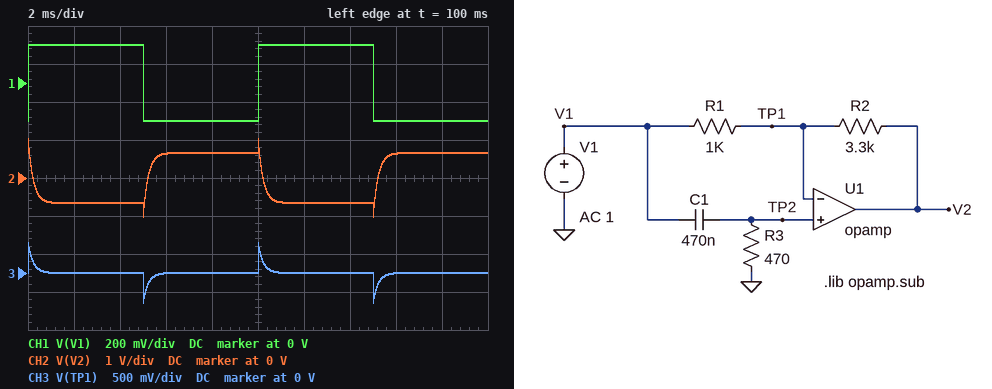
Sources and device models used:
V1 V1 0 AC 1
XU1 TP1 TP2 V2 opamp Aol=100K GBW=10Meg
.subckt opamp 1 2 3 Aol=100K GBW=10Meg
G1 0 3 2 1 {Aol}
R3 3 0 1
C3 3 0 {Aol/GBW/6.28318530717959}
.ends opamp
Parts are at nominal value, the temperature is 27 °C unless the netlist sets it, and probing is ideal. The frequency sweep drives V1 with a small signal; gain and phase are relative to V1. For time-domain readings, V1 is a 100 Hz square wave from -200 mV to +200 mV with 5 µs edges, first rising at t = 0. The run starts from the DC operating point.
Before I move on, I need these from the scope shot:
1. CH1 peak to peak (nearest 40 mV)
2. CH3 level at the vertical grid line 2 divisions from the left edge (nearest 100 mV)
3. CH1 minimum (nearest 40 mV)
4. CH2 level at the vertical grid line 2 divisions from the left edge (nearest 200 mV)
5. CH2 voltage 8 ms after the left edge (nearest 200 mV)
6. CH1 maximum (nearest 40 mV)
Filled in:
400 mV
0 V
-200 mV
-600 mV
600 mV
200 mV
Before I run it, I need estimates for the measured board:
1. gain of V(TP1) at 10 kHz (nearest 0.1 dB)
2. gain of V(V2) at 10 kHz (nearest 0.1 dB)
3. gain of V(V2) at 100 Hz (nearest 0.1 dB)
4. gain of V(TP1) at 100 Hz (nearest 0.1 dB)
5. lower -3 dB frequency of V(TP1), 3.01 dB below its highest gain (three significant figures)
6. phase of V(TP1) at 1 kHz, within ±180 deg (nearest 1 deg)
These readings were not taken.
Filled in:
0 dB
0.2 dB
10.3 dB
-17.2 dB
720 Hz
36 deg
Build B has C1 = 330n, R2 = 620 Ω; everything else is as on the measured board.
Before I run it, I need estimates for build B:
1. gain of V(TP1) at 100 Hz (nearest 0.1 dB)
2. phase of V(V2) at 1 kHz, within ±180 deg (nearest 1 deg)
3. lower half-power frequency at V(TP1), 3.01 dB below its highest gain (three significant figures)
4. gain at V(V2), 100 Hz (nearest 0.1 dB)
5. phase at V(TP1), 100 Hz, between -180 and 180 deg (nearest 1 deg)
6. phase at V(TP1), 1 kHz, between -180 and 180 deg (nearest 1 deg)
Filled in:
-20.3 dB
78 deg
1.03 kHz
-4.1 dB
84 deg
46 deg
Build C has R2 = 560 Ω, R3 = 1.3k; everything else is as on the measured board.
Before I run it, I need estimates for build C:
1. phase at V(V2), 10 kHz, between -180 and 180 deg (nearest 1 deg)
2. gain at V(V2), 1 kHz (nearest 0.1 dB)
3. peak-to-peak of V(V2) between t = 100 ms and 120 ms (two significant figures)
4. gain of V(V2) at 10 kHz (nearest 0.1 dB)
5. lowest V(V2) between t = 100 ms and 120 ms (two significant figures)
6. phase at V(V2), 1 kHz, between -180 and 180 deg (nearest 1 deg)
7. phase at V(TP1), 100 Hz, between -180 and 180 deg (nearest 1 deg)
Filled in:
2 deg
-0.2 dB
1.0 V
0 dB
-510 mV
23 deg
69 deg
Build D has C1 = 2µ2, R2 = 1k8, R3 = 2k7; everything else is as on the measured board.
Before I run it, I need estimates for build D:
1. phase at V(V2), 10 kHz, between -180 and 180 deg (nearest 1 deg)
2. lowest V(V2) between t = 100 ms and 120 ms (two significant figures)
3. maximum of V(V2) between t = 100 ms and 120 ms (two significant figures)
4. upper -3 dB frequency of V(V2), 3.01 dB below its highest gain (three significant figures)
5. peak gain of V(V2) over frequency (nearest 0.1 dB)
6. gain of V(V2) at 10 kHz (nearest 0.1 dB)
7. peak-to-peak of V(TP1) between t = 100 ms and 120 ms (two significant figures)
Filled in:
0 deg
-420 mV
420 mV
43.3 Hz
5.1 dB
0 dB
560 mV
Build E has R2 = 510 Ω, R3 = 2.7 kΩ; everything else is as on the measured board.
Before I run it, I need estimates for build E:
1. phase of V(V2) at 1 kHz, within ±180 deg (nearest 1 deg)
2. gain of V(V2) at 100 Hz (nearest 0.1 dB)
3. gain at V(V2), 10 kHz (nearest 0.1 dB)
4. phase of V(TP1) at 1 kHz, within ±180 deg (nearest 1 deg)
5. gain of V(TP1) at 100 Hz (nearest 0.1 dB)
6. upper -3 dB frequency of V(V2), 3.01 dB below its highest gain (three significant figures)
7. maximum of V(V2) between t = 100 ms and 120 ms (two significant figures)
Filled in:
11 deg
-2.6 dB
0 dB
7 deg
-4.1 dB
6.62 MHz
490 mV
